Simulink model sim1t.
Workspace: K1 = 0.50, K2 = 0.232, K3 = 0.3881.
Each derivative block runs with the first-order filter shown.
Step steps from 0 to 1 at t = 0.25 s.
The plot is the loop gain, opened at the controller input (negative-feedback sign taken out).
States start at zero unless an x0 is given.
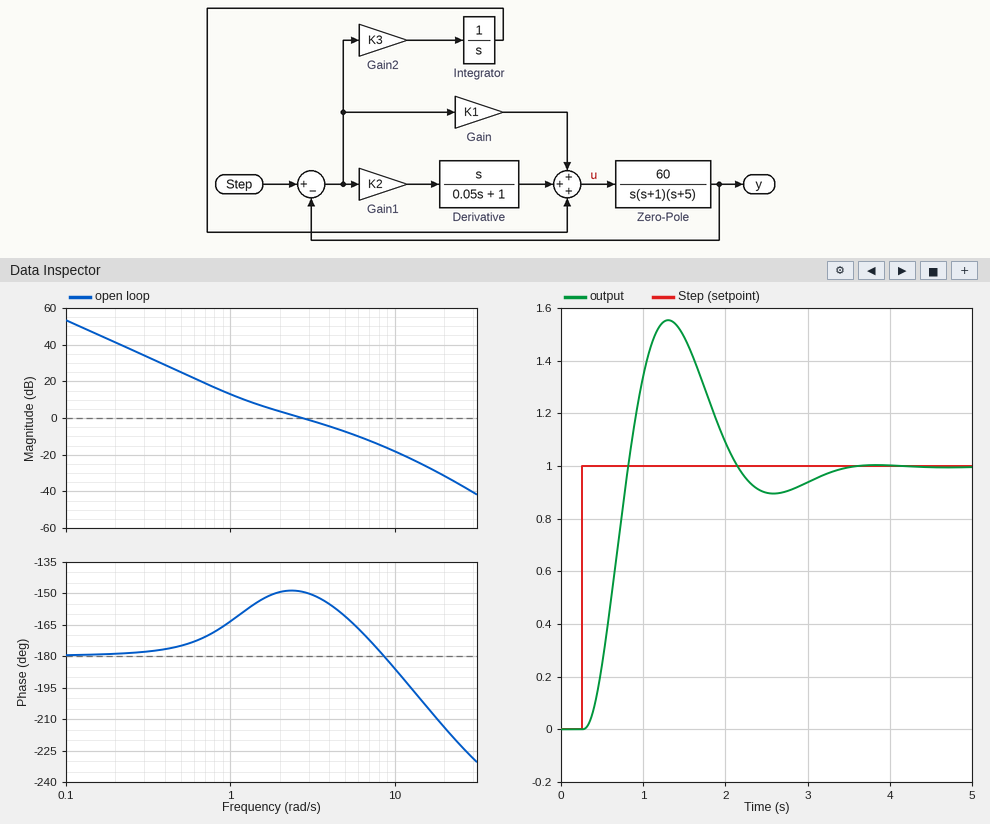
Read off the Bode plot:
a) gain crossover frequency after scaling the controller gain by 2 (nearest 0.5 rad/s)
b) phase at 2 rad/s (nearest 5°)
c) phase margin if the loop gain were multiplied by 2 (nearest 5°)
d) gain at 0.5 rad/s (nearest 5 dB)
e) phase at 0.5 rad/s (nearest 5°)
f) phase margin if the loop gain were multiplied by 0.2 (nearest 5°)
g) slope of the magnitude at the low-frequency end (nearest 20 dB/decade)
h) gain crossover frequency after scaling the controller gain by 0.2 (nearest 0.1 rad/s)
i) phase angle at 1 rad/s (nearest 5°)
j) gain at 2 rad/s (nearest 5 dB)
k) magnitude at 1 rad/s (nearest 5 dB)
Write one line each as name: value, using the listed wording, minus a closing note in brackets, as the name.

gain crossover frequency after scaling the controller gain by 2: 4.5 rad/s
phase at 2 rad/s: -150°
phase margin if the loop gain were multiplied by 2: 20°
gain at 0.5 rad/s: 25 dB
phase at 0.5 rad/s: -175°
phase margin if the loop gain were multiplied by 0.2: 15°
slope of the magnitude at the low-frequency end: -40 dB/decade
gain crossover frequency after scaling the controller gain by 0.2: 0.9 rad/s
phase angle at 1 rad/s: -165°
gain at 2 rad/s: 5 dB
magnitude at 1 rad/s: 15 dB
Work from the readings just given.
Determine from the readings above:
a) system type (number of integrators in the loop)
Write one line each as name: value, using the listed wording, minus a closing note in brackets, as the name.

system type: 2
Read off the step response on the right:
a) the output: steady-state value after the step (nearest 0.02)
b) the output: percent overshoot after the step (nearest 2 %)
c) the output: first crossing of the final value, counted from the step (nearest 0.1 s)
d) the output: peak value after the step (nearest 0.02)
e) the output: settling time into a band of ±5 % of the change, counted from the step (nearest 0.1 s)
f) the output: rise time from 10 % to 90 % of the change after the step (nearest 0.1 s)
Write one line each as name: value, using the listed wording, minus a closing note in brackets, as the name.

the output: steady-state value after the step: 1.00
the output: percent overshoot after the step: 56 %
the output: first crossing of the final value, counted from the step: 0.6 s
the output: peak value after the step: 1.56
the output: settling time into a band of ±5 % of the change, counted from the step: 2.8 s
the output: rise time from 10 % to 90 % of the change after the step: 0.4 s
